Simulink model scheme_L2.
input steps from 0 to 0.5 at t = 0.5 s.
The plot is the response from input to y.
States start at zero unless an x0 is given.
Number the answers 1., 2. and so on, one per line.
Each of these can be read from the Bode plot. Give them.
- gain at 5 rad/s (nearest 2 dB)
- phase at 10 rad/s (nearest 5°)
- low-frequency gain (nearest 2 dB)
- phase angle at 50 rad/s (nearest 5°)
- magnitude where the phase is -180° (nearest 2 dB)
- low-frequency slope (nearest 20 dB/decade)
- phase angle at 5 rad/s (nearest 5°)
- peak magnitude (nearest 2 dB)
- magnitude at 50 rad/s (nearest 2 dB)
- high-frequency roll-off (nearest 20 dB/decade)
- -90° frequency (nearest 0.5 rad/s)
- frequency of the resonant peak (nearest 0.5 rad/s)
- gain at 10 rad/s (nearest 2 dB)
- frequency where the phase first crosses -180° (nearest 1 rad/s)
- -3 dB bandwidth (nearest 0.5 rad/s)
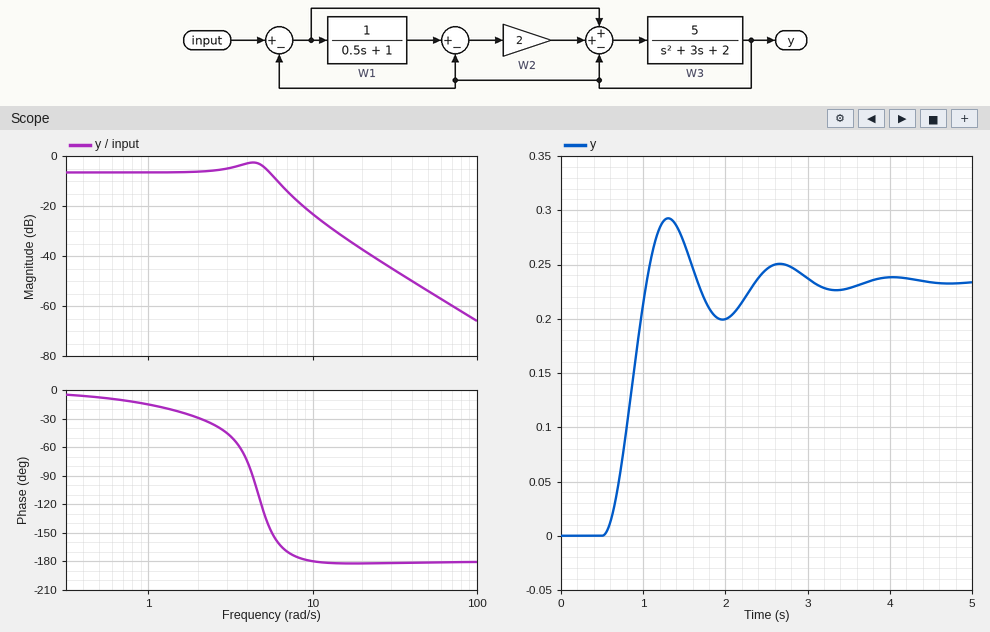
1. -4 dB
2. -180°
3. -6 dB
4. -180°
5. -24 dB
6. 0 dB/decade
7. -125°
8. -2 dB
9. -54 dB
10. -40 dB/decade
11. 4.5 rad/s
12. 4.5 rad/s
13. -24 dB
14. 10 rad/s
15. 6.0 rad/s
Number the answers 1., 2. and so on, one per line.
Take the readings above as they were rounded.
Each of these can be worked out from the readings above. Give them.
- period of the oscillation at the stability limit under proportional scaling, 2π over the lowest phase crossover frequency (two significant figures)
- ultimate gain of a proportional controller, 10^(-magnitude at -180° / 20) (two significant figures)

1. 0.63 s
2. 16
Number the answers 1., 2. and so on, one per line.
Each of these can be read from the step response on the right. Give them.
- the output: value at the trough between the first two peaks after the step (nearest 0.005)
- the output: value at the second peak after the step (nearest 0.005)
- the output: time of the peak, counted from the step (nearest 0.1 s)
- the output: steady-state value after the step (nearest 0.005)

1. 0.200
2. 0.250
3. 0.8 s
4. 0.235
